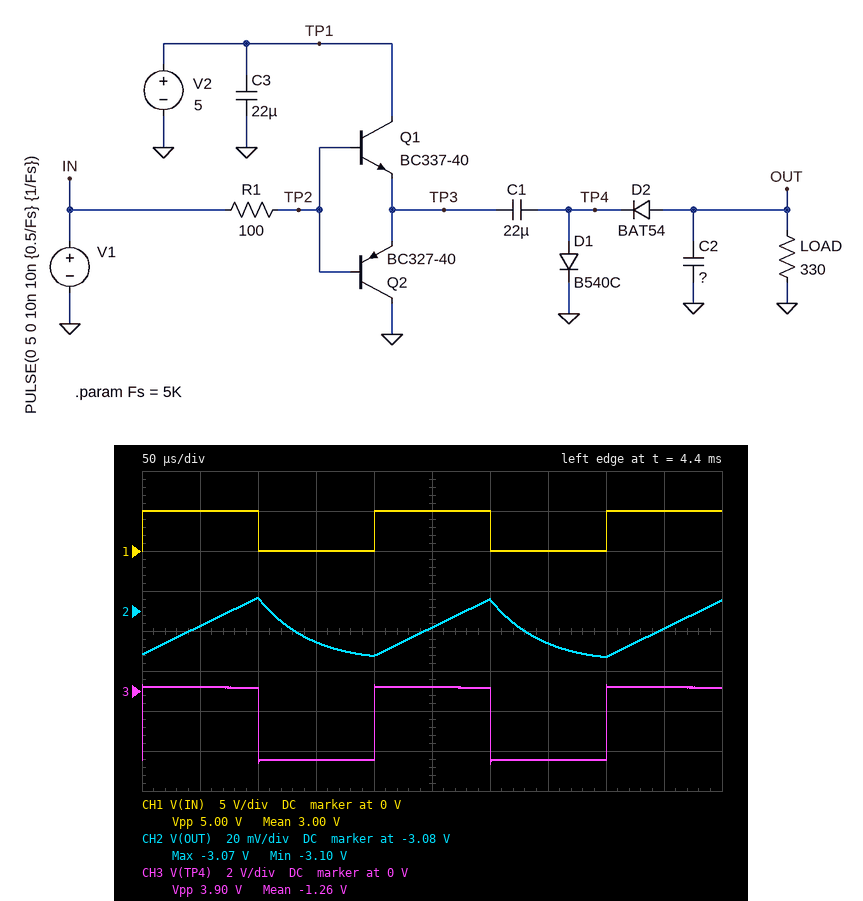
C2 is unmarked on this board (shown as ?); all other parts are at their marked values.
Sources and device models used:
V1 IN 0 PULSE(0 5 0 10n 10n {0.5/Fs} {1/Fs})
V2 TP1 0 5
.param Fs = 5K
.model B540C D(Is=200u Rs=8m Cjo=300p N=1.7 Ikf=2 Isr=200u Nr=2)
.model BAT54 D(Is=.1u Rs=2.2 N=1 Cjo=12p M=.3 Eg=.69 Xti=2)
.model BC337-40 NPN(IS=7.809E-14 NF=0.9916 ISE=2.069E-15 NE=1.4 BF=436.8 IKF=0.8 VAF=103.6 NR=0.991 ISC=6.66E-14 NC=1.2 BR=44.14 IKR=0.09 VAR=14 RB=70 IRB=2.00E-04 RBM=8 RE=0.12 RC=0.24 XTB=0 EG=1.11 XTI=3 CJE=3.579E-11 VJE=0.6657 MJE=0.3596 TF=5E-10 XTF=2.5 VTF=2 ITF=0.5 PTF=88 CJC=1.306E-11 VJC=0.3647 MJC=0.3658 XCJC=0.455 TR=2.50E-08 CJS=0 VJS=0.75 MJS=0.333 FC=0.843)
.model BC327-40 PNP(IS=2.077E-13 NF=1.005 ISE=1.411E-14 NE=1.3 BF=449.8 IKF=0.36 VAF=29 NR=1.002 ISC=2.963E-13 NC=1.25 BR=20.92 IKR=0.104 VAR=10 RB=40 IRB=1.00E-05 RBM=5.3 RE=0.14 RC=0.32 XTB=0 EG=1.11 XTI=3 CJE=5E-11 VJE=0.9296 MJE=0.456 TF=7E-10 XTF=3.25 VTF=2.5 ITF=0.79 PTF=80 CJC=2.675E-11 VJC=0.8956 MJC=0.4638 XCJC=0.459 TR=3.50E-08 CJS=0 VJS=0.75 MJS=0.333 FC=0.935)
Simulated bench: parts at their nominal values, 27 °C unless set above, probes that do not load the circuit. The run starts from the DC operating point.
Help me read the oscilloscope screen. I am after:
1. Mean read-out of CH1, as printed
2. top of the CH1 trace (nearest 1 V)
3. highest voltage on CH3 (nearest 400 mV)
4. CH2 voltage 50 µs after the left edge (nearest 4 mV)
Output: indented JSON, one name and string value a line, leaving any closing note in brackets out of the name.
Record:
{
  "Mean read-out of CH1, as printed": "3.00 V",
  "top of the CH1 trace": "5 V",
  "highest voltage on CH3": "400 mV",
  "CH2 voltage 50 µs after the left edge": "-3.088 V"
}
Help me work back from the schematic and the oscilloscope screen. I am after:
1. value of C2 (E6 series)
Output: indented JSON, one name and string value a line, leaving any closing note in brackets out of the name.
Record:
{
  "value of C2": "33 µF"
}
